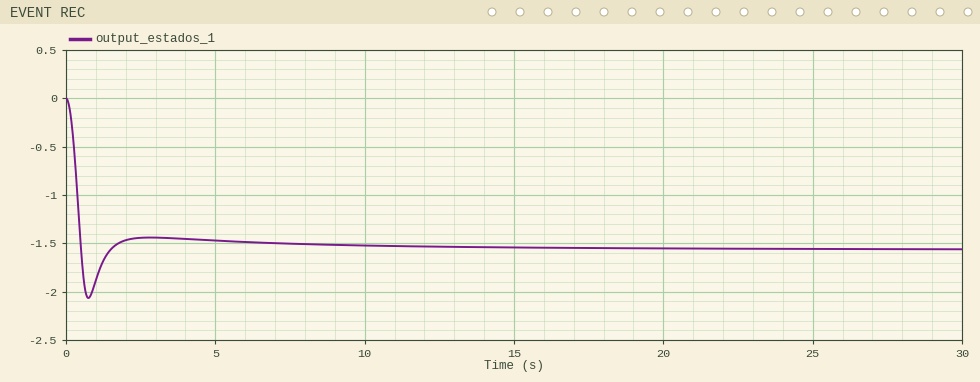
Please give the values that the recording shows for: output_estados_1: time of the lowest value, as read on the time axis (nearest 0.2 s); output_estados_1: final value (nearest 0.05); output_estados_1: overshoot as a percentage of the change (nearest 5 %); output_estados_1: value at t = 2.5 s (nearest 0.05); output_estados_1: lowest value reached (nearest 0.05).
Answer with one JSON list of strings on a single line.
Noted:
["0.8 s", "-1.55", "30 %", "-1.45", "-2.05"]
